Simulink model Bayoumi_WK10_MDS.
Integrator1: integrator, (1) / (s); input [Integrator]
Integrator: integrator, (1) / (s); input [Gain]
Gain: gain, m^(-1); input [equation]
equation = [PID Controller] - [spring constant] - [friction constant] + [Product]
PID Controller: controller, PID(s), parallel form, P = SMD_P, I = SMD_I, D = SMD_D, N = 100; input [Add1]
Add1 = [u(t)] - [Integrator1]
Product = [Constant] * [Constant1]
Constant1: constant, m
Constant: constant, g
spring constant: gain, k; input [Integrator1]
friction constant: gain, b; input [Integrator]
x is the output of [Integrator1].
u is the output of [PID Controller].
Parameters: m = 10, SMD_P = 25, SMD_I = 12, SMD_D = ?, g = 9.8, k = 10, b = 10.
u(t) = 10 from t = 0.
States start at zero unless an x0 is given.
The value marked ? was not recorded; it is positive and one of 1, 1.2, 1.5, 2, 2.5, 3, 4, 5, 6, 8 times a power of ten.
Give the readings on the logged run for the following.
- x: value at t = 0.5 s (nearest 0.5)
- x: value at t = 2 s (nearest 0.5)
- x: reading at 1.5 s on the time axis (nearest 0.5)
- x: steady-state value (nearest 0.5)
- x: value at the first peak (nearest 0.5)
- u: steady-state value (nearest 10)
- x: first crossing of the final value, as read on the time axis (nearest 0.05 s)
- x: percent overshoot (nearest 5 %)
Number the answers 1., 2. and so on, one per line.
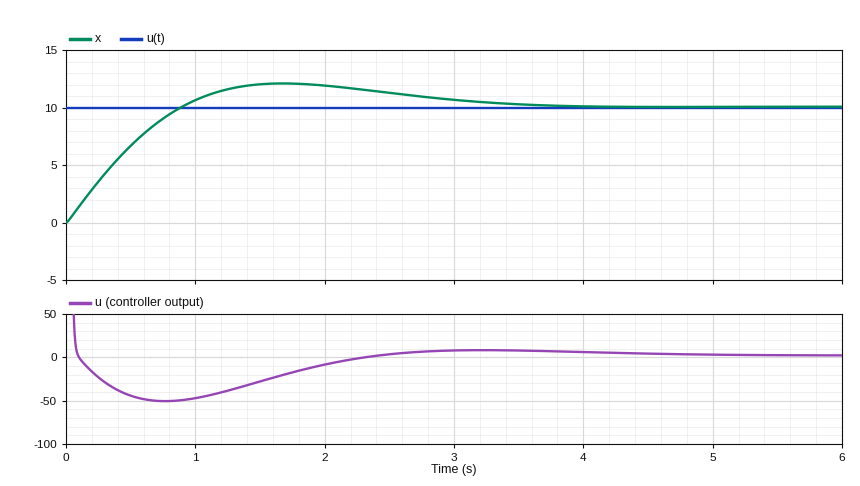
1. 6.5
2. 12.0
3. 12.0
4. 10.0
5. 12.0
6. 0
7. 0.90 s
8. 20 %
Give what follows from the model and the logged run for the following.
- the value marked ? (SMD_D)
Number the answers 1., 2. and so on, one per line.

1. 15
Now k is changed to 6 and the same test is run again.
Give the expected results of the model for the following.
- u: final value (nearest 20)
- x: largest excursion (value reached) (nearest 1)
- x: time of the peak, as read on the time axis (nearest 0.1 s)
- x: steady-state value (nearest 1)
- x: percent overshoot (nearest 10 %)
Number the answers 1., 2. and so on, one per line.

1. -40
2. 13
3. 1.8 s
4. 10
5. 30 %
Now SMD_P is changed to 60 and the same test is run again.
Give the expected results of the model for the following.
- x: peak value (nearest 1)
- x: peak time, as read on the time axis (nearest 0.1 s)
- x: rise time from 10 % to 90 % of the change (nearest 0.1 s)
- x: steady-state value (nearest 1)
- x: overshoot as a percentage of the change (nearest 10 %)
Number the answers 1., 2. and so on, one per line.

1. 13
2. 1.1 s
3. 0.5 s
4. 10
5. 30 %
